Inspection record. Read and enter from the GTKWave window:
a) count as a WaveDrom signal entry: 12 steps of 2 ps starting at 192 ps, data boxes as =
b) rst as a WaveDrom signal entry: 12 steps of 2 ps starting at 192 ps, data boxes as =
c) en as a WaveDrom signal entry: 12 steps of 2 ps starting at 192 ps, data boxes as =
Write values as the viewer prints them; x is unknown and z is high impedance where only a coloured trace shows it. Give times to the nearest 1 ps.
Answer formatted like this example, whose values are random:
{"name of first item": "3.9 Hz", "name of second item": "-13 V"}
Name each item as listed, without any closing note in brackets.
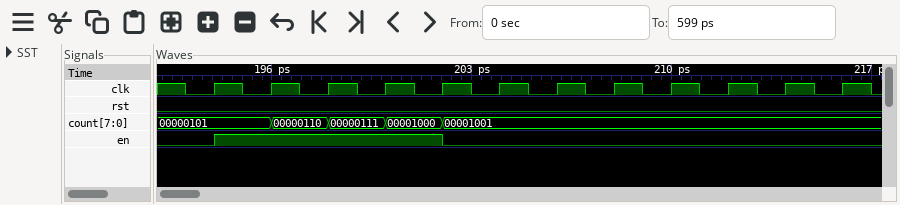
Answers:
{"count as a WaveDrom signal entry: 12 steps of 2 ps starting at 192 ps, data boxes as =": "{name: 'count', wave: '=.====......', data: '00000101 00000110 00000111 00001000 00001001'}", "rst as a WaveDrom signal entry: 12 steps of 2 ps starting at 192 ps, data boxes as =": "{name: 'rst', wave: '0...........'}", "en as a WaveDrom signal entry: 12 steps of 2 ps starting at 192 ps, data boxes as =": "{name: 'en', wave: '01...0......'}"}
